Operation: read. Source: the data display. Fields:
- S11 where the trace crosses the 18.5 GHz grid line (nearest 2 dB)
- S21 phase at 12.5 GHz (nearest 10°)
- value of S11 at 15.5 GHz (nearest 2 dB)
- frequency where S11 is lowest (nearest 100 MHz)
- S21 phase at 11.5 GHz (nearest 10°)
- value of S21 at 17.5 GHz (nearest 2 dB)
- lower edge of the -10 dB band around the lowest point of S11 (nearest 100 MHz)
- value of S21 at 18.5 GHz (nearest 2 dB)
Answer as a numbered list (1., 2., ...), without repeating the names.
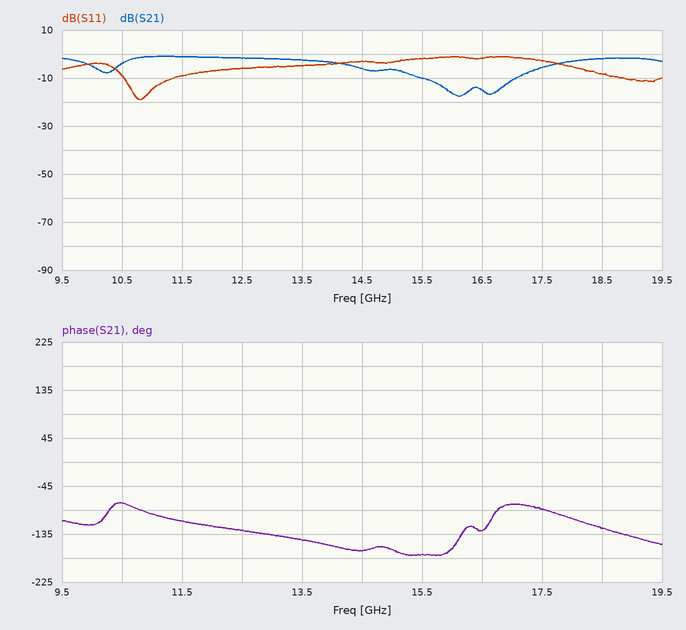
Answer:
1. -8 dB
2. -130°
3. -2 dB
4. 10.8 GHz
5. -110°
6. -6 dB
7. 10.5 GHz
8. -2 dB
